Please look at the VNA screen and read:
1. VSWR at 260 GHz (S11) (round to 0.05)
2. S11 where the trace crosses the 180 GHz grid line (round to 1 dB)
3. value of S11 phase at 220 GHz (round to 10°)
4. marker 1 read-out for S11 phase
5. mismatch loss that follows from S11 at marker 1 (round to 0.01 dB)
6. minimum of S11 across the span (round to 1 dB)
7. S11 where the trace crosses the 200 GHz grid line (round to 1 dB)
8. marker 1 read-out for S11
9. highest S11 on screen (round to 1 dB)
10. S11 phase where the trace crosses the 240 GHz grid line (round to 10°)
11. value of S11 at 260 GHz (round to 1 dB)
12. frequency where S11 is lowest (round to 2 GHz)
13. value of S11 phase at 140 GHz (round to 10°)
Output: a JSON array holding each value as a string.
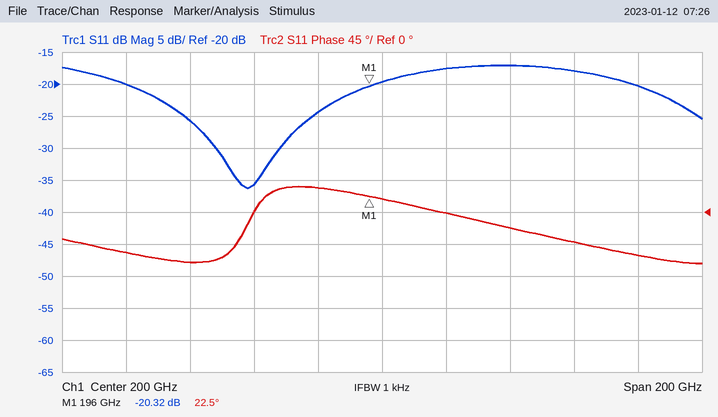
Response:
["1.30", "-24 dB", "0°", "22.5°", "0.04 dB", "-36 dB", "-20 dB", "-20.32 dB", "-17 dB", "-20°", "-18 dB", "158 GHz", "-70°"]
